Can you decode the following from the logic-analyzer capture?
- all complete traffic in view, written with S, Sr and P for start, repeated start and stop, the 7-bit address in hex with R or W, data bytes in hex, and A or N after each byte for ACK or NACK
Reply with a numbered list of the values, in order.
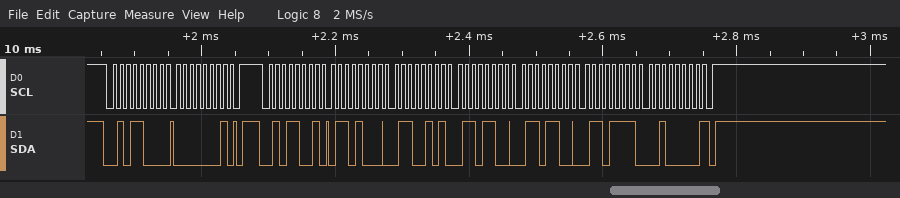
1. S 2CW A 01 A P S 2CR A 68 A 65 A 6C A 6C A 6F A 20 N P
